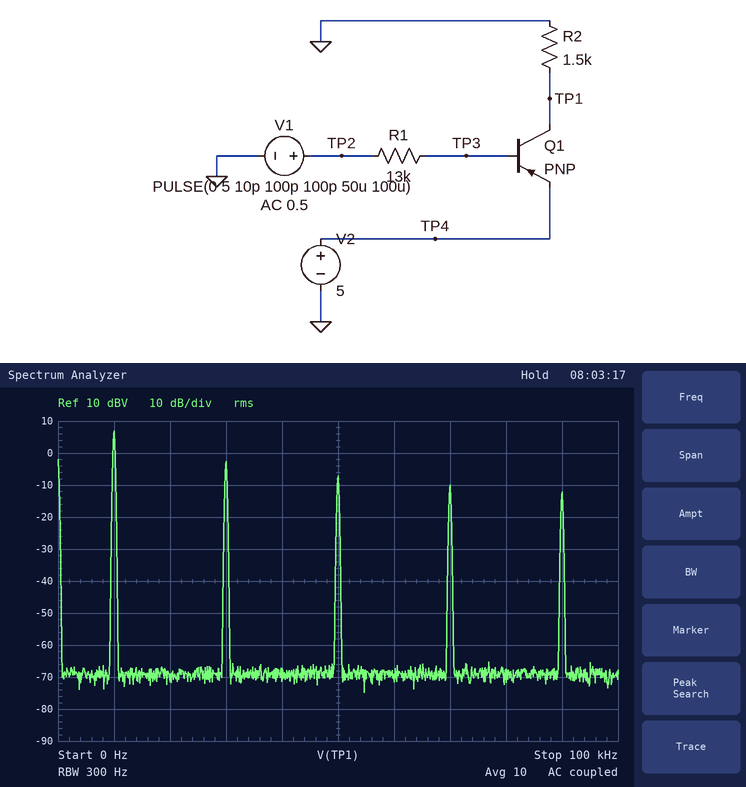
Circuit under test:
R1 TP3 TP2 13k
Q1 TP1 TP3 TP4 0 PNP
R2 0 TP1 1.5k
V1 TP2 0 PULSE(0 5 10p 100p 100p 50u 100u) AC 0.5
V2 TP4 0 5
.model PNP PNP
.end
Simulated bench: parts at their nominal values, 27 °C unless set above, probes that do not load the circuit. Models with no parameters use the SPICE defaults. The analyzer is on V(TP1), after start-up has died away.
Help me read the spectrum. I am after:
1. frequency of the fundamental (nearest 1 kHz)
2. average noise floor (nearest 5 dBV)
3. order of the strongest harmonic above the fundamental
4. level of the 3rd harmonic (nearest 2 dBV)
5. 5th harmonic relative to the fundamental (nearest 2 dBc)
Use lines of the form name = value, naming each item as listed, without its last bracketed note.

frequency of the fundamental = 10 kHz
average noise floor = -70 dBV
order of the strongest harmonic above the fundamental = 3
level of the 3rd harmonic = -2 dBV
5th harmonic relative to the fundamental = -14 dBc
